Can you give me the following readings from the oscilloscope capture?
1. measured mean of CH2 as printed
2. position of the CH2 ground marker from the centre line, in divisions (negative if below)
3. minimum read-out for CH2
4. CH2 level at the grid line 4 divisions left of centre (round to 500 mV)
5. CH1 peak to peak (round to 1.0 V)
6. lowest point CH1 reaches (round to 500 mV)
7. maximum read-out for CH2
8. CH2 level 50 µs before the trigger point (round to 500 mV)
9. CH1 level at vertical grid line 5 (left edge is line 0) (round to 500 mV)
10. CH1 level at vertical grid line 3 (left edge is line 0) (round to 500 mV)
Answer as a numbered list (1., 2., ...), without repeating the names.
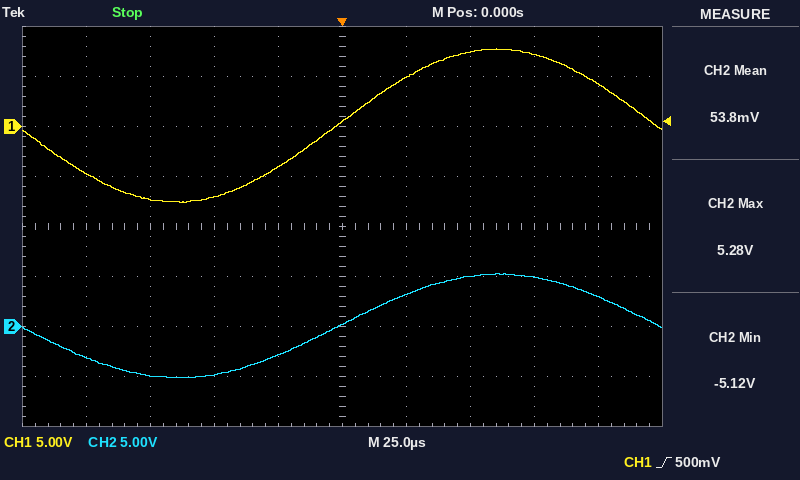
1. 53.8 mV
2. -2.0 div
3. -5.12 V
4. -3.0 V
5. 15.0 V
6. -7.5 V
7. 5.28 V
8. -5.0 V
9. 500 mV
10. -7.0 V
